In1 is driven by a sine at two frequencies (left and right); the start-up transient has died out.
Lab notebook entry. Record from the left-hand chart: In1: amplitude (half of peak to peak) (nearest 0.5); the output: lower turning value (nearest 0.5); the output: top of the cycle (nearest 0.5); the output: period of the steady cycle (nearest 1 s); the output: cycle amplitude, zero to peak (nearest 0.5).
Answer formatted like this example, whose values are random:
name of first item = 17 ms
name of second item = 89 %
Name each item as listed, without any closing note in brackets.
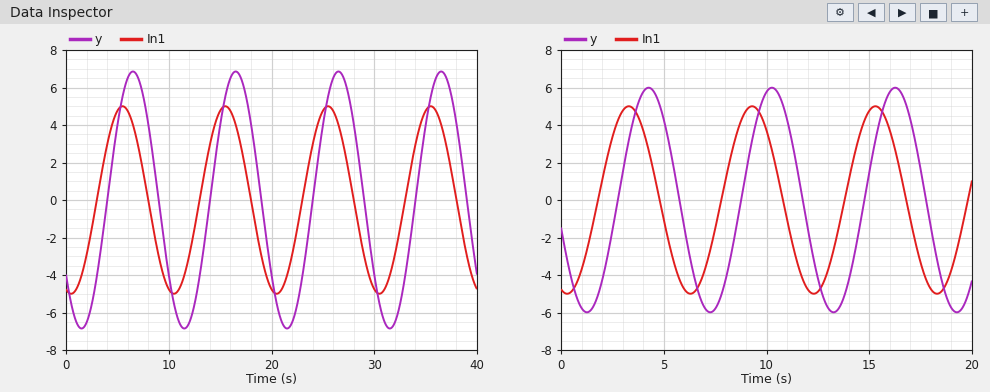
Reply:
In1: amplitude (half of peak to peak) = 5.0
the output: lower turning value = -7.0
the output: top of the cycle = 7.0
the output: period of the steady cycle = 10 s
the output: cycle amplitude, zero to peak = 7.0
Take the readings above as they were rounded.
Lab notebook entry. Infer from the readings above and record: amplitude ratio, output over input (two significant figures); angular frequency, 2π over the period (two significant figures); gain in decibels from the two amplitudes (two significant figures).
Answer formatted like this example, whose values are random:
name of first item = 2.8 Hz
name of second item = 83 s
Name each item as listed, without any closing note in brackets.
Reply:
amplitude ratio, output over input = 1.4
angular frequency, 2π over the period = 0.63 rad/s
gain in decibels from the two amplitudes = 2.9 dB
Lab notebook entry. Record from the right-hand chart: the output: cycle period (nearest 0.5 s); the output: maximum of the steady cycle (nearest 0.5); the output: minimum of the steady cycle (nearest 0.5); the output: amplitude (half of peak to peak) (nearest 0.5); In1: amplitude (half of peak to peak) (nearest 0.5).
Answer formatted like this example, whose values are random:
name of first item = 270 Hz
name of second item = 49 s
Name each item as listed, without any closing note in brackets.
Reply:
the output: cycle period = 6.0 s
the output: maximum of the steady cycle = 6.0
the output: minimum of the steady cycle = -6.0
the output: amplitude (half of peak to peak) = 6.0
In1: amplitude (half of peak to peak) = 5.0
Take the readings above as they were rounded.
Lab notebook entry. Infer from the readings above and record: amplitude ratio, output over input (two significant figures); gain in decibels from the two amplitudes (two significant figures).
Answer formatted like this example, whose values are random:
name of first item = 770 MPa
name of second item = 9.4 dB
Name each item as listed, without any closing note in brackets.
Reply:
amplitude ratio, output over input = 1.2
gain in decibels from the two amplitudes = 1.6 dB
